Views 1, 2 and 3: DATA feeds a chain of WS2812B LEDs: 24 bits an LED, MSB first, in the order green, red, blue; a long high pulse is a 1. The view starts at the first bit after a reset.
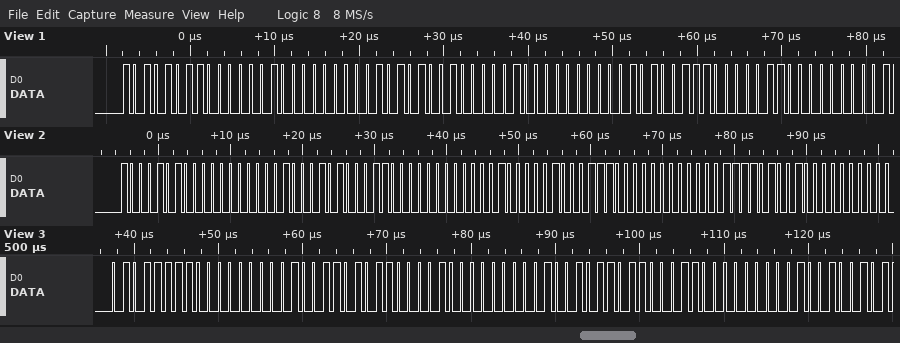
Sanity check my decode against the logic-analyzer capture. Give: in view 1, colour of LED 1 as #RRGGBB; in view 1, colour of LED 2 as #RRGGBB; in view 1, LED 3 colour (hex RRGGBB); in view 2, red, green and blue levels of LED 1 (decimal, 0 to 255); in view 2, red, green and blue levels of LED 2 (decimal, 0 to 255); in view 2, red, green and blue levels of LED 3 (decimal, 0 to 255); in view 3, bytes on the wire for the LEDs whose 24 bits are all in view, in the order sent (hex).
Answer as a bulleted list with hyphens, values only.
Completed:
- #02AB00
- #04A900
- #06A700
- 0, 138, 34
- 0, 140, 32
- 0, 142, 30
- 5F 00 4D 61 00 4B 63 00 49
